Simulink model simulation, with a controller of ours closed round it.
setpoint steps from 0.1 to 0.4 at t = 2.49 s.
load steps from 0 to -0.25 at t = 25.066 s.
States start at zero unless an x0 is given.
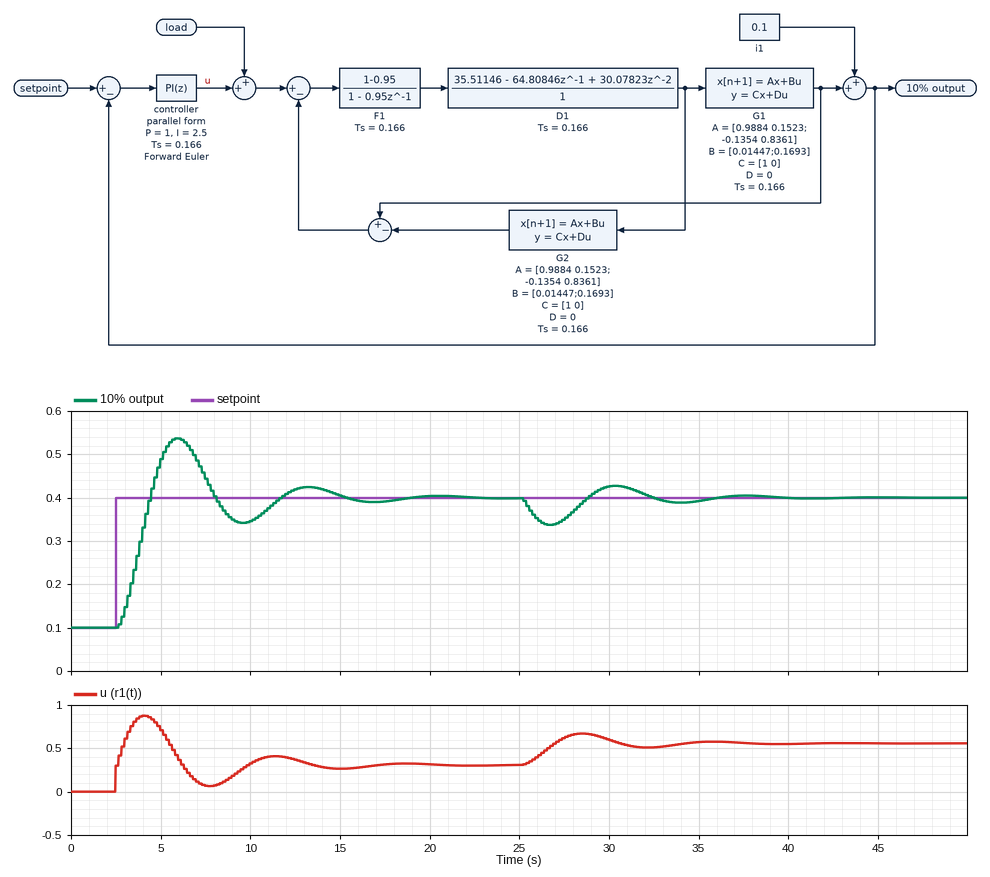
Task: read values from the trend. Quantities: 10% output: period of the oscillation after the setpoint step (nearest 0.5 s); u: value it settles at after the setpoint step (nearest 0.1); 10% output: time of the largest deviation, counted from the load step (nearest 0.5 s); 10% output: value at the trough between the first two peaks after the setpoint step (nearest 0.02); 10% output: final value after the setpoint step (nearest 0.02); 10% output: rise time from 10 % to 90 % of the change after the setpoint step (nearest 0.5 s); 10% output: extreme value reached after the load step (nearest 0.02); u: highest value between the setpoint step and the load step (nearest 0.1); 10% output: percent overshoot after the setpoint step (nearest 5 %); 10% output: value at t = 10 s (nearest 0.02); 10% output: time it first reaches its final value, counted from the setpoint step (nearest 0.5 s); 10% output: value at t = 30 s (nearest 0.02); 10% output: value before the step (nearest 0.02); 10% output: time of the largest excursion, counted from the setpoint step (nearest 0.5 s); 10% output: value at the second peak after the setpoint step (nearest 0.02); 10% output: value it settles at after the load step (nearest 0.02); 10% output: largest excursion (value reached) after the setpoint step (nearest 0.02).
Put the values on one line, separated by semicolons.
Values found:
7.5 s; 0.3; 1.5 s; 0.34; 0.40; 1.5 s; 0.34; 0.9; 45 %; 0.34; 2.0 s; 0.42; 0.10; 3.5 s; 0.42; 0.40; 0.54
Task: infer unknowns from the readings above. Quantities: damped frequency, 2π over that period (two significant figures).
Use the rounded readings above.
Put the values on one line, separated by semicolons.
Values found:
0.84 rad/s
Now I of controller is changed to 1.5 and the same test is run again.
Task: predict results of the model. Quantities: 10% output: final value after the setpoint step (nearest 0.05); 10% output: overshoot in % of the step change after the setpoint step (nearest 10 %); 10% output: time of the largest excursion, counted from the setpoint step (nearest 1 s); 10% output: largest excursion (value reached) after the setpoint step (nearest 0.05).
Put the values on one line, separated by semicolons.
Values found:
0.40; 30 %; 4 s; 0.50
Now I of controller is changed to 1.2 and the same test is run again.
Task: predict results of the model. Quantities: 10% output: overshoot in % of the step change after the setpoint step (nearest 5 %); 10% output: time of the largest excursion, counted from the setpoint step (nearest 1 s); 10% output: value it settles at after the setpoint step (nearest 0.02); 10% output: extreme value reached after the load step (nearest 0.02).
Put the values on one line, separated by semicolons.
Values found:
25 %; 5 s; 0.40; 0.32
